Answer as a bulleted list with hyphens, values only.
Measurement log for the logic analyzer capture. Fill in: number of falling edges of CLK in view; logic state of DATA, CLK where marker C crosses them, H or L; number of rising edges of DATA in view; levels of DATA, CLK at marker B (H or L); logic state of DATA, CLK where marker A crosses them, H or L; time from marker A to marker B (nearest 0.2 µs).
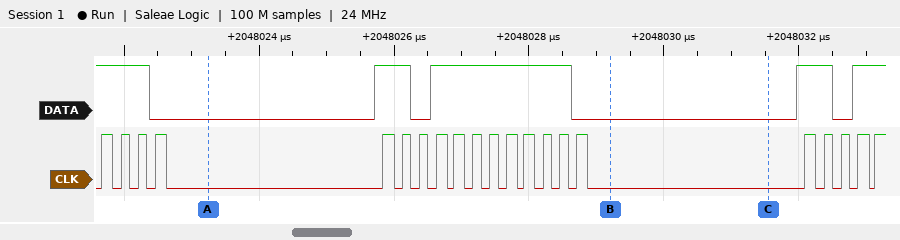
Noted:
- 20
- DATA=L, CLK=L
- 4
- DATA=L, CLK=L
- DATA=L, CLK=L
- 6 µs
